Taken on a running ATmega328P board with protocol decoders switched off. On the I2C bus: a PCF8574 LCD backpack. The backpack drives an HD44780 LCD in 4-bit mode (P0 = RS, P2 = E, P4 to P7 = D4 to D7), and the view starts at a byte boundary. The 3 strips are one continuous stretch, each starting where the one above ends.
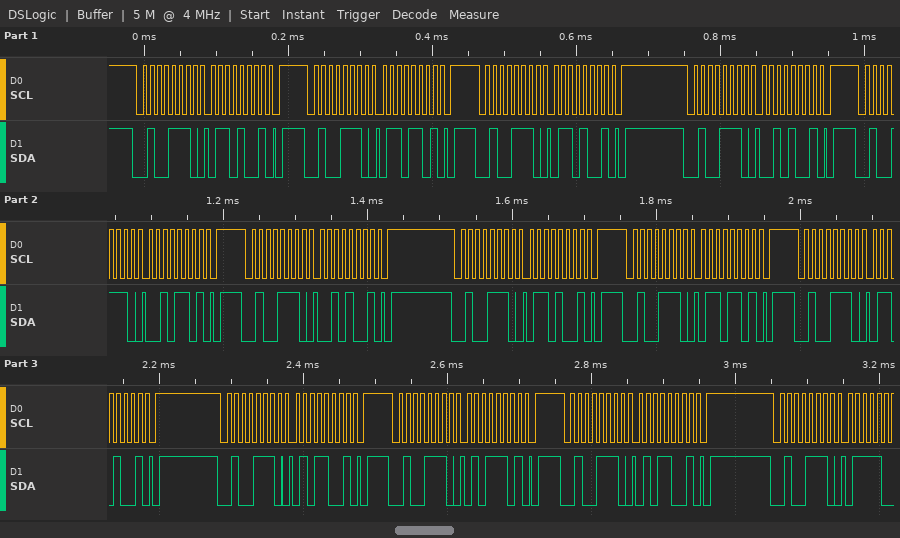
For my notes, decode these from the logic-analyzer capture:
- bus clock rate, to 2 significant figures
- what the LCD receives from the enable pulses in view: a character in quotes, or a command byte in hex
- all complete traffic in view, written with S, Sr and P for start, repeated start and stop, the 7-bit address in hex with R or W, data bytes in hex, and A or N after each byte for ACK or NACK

100 kHz
'b' 'e'
S 27W A 69 A P S 27W A 6D A P S 27W A 69 A P S 27W A 29 A P S 27W A 2D A P S 27W A 29 A P S 27W A 69 A P S 27W A 6D A P S 27W A 69 A P S 27W A 59 A P S 27W A 5D A P S 27W A 59 A P S 27W A
